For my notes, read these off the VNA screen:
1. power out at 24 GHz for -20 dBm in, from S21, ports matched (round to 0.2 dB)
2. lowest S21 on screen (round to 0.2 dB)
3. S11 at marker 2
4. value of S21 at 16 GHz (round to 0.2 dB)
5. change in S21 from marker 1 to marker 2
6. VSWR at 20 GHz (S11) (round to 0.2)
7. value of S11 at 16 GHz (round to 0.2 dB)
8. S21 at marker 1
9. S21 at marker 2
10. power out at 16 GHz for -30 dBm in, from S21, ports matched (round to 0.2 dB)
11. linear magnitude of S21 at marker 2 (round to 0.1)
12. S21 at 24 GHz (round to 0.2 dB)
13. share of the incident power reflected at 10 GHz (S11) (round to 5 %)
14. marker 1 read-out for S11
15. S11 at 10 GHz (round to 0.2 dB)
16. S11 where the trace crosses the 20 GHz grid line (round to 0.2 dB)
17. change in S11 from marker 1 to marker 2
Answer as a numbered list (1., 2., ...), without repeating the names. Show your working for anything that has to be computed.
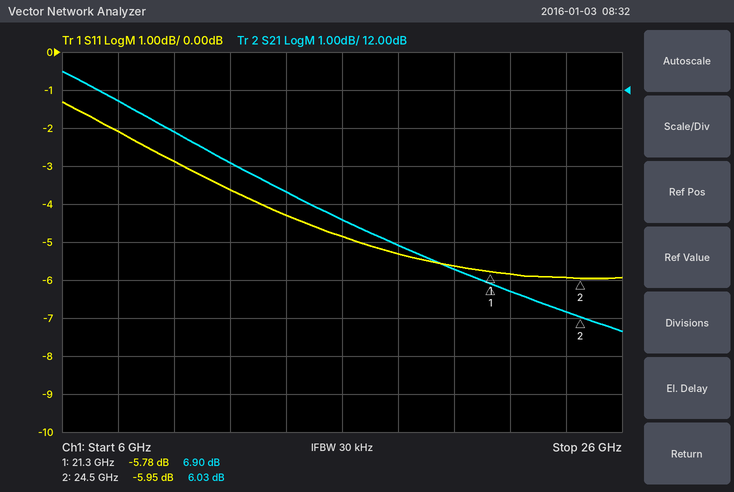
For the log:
1. -20 dBm + (6.2 dB) = -13.8 dBm
2. 5.6 dB
3. -5.95 dB
4. 8.6 dB
5. 6.03 − (6.9) = -0.87 dB
6. |Γ| = 10^(-5.6/20) = 0.5248; VSWR = (1 + 0.5248)/(1 − 0.5248) ≈ 3.2
7. -4.8 dB
8. 6.90 dB
9. 6.03 dB
10. -30 dBm + (8.6 dB) = -21.4 dBm
11. 10^(6.03/20) ≈ 2.0
12. 6.2 dB
13. 10^(-2.8/10) ≈ 52.5 %, so 50 % to the nearest 5 %
14. -5.78 dB
15. -2.8 dB
16. -5.6 dB
17. -5.95 − (-5.78) = -0.17 dB
